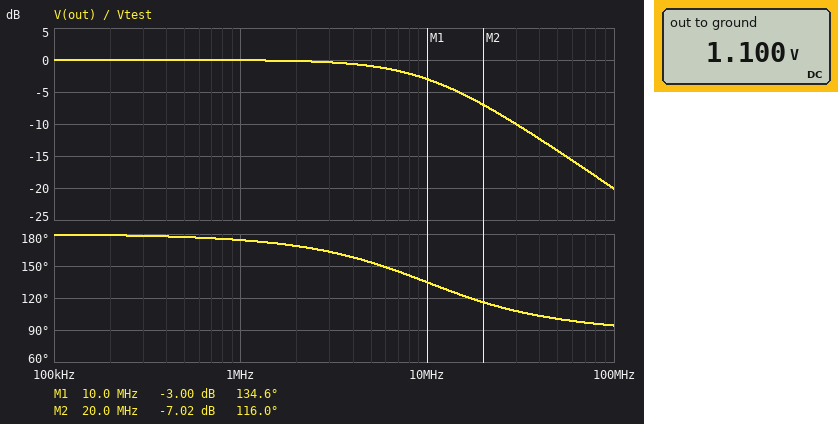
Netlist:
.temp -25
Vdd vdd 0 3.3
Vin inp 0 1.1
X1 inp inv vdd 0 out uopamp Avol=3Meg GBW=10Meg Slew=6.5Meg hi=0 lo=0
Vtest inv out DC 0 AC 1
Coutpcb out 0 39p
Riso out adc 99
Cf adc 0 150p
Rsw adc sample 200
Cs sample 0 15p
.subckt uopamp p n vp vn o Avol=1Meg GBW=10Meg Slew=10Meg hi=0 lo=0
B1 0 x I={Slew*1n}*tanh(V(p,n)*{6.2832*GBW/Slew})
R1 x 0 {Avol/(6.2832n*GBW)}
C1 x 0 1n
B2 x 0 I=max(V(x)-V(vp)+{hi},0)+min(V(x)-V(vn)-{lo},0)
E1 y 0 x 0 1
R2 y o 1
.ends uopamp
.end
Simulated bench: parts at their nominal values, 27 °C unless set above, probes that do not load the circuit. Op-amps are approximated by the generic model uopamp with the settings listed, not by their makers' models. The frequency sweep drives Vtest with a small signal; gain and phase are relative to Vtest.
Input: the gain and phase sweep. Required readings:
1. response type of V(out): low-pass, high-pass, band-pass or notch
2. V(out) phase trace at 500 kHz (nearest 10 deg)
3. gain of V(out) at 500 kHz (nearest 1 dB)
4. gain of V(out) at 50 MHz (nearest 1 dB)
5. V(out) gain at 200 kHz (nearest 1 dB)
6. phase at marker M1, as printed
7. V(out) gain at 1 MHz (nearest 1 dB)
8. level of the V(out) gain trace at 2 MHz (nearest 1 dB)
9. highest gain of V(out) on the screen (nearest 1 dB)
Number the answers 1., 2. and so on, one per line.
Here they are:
1. low-pass
2. 180 deg
3. 0 dB
4. -14 dB
5. 0 dB
6. 134.6 deg
7. 0 dB
8. 0 dB
9. 0 dB
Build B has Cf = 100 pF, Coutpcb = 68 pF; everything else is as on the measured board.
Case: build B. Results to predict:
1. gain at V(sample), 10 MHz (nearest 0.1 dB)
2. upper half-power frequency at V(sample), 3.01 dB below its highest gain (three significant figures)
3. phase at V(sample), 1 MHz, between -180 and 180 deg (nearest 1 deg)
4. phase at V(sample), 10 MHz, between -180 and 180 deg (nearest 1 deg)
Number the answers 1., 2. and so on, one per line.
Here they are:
1. -5.0 dB
2. 7.29 MHz
3. 169 deg
4. 89 deg
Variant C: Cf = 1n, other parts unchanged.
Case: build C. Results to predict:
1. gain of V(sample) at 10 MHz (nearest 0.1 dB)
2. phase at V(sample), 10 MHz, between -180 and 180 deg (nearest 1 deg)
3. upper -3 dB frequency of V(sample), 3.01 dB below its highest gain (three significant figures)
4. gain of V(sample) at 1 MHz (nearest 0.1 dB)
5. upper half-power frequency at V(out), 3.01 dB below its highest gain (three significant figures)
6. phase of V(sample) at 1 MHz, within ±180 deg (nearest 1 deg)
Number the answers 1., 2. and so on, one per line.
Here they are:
1. -19.3 dB
2. 43 deg
3. 1.55 MHz
4. -1.5 dB
5. 9.94 MHz
6. 141 deg
